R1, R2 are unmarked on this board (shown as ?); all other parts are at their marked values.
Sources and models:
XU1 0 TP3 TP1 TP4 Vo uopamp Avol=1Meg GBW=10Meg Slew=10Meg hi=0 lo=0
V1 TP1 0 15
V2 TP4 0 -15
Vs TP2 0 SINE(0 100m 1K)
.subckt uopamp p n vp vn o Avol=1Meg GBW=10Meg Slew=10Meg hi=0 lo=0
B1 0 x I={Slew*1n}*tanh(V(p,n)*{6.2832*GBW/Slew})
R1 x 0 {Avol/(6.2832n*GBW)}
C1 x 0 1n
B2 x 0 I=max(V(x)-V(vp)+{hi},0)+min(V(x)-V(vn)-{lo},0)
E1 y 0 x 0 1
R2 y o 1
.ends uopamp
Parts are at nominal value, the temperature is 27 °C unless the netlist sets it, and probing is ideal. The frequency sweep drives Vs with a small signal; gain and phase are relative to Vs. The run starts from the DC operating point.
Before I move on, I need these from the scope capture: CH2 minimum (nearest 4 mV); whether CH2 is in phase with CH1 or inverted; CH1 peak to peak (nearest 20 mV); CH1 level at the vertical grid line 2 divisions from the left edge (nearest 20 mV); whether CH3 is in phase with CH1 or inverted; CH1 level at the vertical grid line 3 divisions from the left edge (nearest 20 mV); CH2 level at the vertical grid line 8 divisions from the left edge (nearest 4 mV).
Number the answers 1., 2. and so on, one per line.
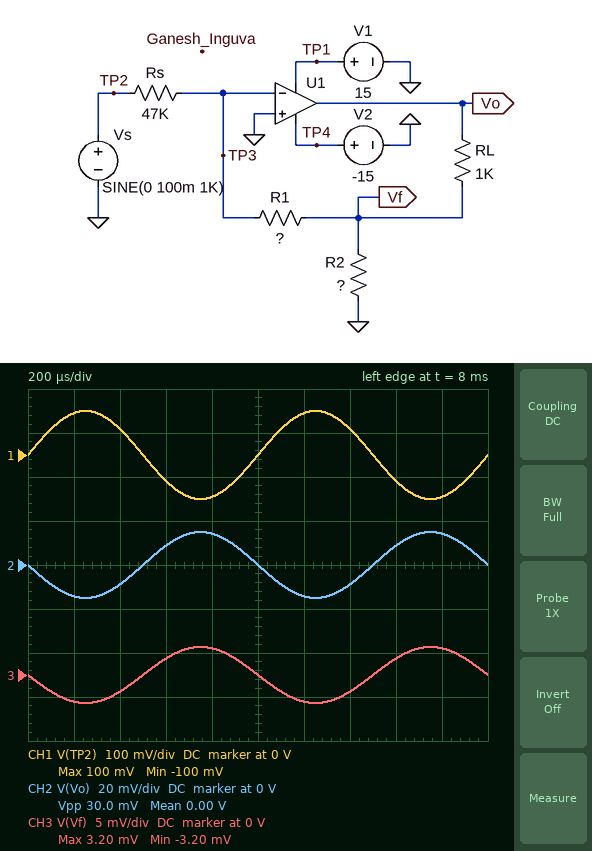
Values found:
1. -16 mV
2. inverted
3. 200 mV
4. 60 mV
5. inverted
6. -60 mV
7. 8 mV
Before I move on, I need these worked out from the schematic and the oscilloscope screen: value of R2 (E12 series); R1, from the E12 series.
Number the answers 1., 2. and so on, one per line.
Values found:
1. 330 Ω
2. 1.5 kΩ
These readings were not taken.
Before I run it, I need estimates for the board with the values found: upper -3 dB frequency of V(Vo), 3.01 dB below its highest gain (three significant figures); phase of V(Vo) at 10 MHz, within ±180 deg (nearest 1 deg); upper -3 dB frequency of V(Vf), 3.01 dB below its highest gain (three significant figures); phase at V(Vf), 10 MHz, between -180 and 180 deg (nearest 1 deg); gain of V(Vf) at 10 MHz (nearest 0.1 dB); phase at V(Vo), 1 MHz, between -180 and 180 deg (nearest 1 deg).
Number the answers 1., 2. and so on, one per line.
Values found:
1. 2.39 MHz
2. 103 deg
3. 2.45 MHz
4. 70 deg
5. -41.0 dB
6. 157 deg
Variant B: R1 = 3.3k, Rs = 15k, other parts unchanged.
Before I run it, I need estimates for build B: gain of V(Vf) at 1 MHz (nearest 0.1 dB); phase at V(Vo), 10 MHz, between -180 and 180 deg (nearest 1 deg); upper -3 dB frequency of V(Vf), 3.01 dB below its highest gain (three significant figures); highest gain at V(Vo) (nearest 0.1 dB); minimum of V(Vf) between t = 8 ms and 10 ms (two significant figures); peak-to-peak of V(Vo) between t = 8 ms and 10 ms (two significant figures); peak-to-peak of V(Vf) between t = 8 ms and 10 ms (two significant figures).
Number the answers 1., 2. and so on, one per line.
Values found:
1. -14.1 dB
2. 101 deg
3. 2.01 MHz
4. -0.4 dB
5. -22 mV
6. 190 mV
7. 44 mV
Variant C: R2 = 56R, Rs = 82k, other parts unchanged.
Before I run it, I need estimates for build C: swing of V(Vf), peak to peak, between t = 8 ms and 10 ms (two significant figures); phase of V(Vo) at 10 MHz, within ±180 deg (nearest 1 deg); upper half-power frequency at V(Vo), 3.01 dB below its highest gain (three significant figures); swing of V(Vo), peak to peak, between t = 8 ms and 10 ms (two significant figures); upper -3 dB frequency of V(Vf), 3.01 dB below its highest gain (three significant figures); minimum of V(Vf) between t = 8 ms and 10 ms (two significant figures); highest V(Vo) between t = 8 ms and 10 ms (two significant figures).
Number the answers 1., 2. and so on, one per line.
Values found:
1. 3.7 mV
2. 93 deg
3. 520 kHz
4. 71 mV
5. 521 kHz
6. -1.8 mV
7. 36 mV
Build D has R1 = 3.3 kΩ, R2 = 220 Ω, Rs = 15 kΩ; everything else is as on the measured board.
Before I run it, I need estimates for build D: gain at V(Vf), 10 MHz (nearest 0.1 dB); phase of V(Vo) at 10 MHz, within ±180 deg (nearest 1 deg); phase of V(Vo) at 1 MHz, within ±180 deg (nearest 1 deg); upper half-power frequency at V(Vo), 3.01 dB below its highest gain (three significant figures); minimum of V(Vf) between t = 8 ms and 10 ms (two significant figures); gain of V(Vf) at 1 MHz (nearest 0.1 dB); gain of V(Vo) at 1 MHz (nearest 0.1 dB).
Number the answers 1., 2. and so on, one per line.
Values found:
1. -29.6 dB
2. 98 deg
3. 146 deg
4. 1.46 MHz
5. -22 mV
6. -14.8 dB
7. 0.5 dB
